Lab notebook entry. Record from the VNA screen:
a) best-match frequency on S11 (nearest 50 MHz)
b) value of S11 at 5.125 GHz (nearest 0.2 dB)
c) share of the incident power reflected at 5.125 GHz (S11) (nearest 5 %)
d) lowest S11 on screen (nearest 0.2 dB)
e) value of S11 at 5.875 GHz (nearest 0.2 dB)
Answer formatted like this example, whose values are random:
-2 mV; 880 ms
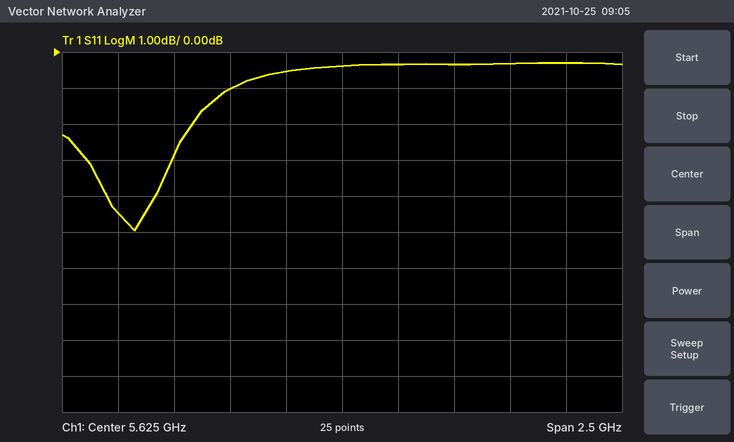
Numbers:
4.70 GHz; -1.0 dB; 80 %; -5.0 dB; -0.4 dB
